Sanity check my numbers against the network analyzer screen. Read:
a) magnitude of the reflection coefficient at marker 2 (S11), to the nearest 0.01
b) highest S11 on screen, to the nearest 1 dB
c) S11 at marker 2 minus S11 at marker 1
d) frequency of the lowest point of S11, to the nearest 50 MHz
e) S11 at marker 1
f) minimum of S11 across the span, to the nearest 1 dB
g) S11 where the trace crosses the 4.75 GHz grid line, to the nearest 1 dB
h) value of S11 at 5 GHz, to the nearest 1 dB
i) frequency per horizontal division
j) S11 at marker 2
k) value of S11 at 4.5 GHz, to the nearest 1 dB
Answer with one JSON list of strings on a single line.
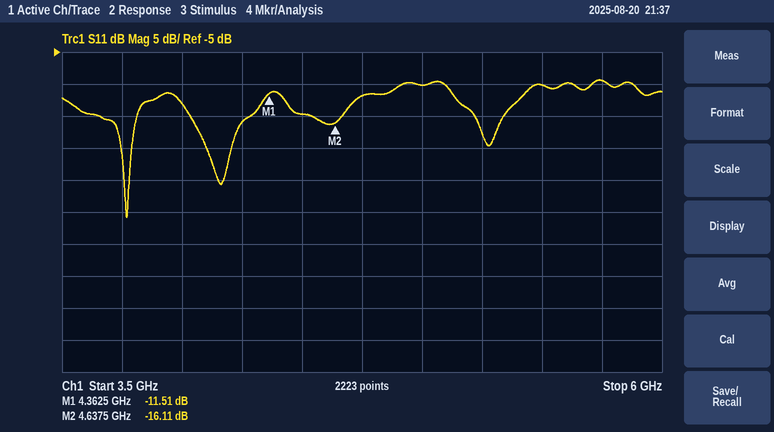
["0.16", "-9 dB", "-4.60 dB", "3.75 GHz", "-11.51 dB", "-31 dB", "-12 dB", "-10 dB", "250 MHz", "-16.11 dB", "-15 dB"]
